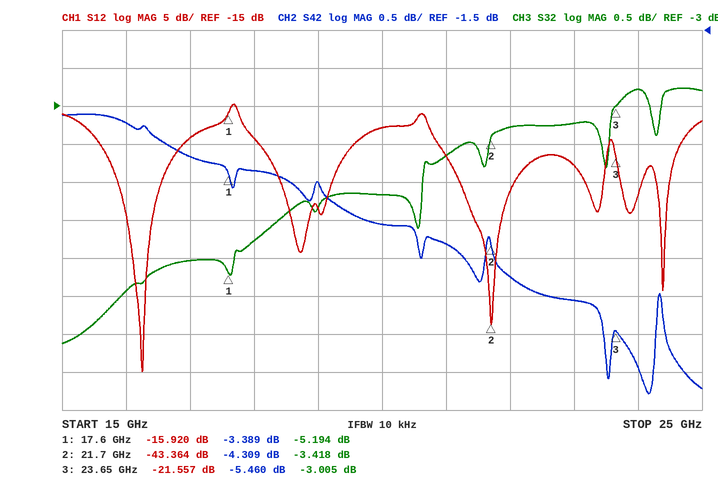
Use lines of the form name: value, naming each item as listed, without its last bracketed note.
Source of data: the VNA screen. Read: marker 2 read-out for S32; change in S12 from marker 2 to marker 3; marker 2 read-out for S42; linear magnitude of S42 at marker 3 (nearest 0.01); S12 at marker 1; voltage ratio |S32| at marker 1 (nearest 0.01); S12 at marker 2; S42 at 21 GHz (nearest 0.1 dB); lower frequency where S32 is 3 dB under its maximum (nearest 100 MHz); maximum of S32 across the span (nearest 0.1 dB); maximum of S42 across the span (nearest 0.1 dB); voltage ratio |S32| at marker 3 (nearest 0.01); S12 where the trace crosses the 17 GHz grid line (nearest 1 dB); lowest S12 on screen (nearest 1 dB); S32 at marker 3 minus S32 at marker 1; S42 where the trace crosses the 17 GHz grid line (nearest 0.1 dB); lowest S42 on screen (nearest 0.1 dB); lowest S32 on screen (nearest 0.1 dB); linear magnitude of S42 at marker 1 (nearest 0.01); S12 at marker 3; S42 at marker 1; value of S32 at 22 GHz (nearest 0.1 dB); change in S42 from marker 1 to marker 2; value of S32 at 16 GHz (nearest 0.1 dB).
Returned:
marker 2 read-out for S32: -3.418 dB
change in S12 from marker 2 to marker 3: 21.807 dB
marker 2 read-out for S42: -4.309 dB
linear magnitude of S42 at marker 3: 0.53
S12 at marker 1: -15.920 dB
voltage ratio |S32| at marker 1: 0.55
S12 at marker 2: -43.364 dB
S42 at 21 GHz: -4.3 dB
lower frequency where S32 is 3 dB under its maximum: 15.6 GHz
maximum of S32 across the span: -2.8 dB
maximum of S42 across the span: -2.6 dB
voltage ratio |S32| at marker 3: 0.71
S12 where the trace crosses the 17 GHz grid line: -19 dB
lowest S12 on screen: -50 dB
S32 at marker 3 minus S32 at marker 1: 2.189 dB
S42 where the trace crosses the 17 GHz grid line: -3.2 dB
lowest S42 on screen: -6.3 dB
lowest S32 on screen: -6.1 dB
linear magnitude of S42 at marker 1: 0.68
S12 at marker 3: -21.557 dB
S42 at marker 1: -3.389 dB
value of S32 at 22 GHz: -3.3 dB
change in S42 from marker 1 to marker 2: -0.920 dB
value of S32 at 16 GHz: -5.4 dB
